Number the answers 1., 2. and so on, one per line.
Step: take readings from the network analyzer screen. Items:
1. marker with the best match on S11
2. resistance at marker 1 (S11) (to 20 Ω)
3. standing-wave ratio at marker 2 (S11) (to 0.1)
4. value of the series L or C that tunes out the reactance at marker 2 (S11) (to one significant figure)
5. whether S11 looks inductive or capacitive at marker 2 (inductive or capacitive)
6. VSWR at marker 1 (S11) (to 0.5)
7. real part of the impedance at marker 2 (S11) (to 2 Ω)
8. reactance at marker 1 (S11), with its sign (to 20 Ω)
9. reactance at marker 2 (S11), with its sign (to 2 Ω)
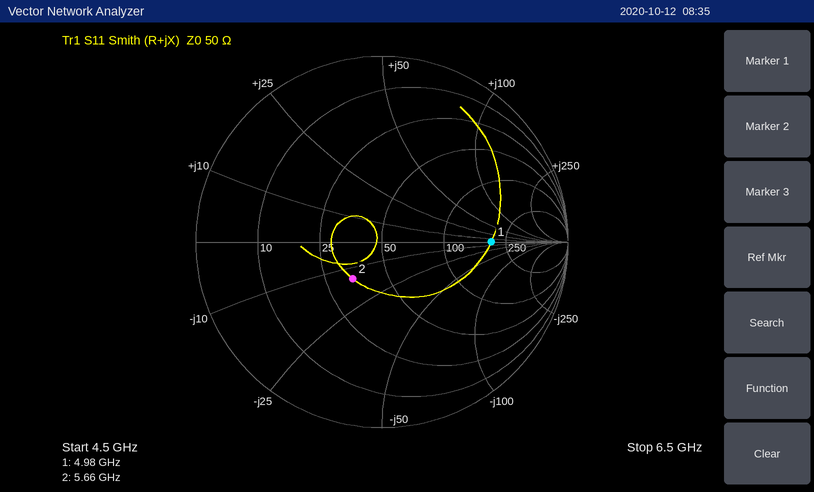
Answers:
1. marker 2
2. 200 Ω
3. 1.7
4. 400 pH
5. capacitive
6. 4.0
7. 34 Ω
8. 0 Ω
9. -14 Ω
